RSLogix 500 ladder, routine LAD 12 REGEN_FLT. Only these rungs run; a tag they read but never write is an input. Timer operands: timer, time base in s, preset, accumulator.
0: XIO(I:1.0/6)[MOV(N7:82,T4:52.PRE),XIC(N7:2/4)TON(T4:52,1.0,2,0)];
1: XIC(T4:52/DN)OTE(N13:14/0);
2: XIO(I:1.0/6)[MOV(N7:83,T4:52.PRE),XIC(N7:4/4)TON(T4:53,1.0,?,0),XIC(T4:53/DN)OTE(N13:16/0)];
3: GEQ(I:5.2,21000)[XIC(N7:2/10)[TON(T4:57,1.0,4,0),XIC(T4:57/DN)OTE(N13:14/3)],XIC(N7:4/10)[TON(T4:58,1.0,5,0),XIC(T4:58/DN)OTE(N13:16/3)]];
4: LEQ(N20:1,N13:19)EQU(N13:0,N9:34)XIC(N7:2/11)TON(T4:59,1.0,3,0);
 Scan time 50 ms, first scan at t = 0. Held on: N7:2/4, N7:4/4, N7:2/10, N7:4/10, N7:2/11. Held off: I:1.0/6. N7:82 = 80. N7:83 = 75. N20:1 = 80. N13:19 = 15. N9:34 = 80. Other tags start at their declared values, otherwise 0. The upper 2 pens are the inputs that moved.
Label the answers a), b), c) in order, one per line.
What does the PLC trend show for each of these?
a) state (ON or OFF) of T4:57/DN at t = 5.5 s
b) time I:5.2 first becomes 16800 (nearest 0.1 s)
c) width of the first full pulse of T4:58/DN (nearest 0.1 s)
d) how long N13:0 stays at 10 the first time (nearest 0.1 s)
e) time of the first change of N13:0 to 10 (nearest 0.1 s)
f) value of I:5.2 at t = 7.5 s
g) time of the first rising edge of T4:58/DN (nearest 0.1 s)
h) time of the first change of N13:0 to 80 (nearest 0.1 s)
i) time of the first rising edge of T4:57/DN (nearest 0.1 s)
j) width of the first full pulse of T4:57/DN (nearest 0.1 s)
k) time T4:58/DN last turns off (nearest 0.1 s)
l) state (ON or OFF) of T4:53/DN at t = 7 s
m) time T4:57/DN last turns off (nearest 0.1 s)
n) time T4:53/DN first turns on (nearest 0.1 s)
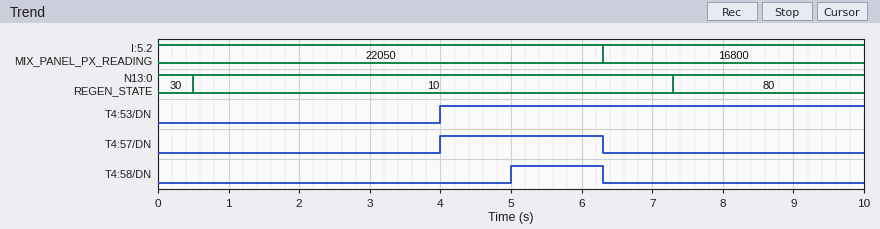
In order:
a) ON
b) 6.3 s
c) 1.3 s
d) 6.8 s
e) 0.5 s
f) 16800
g) 5.0 s
h) 7.3 s
i) 4.0 s
j) 2.3 s
k) 6.3 s
l) ON
m) 6.3 s
n) 4.0 s
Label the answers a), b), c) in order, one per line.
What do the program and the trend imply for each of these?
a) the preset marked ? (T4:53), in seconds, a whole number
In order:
a) 4 s
